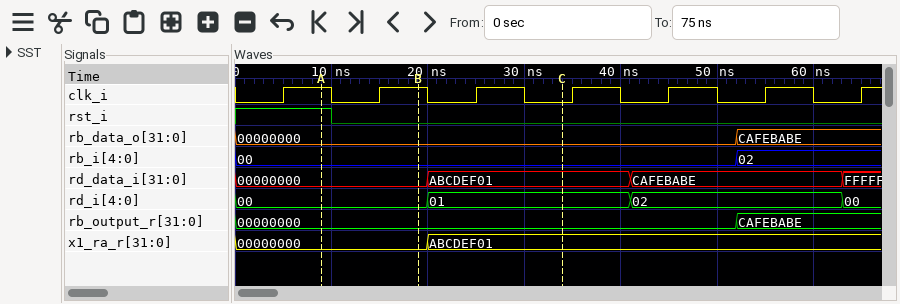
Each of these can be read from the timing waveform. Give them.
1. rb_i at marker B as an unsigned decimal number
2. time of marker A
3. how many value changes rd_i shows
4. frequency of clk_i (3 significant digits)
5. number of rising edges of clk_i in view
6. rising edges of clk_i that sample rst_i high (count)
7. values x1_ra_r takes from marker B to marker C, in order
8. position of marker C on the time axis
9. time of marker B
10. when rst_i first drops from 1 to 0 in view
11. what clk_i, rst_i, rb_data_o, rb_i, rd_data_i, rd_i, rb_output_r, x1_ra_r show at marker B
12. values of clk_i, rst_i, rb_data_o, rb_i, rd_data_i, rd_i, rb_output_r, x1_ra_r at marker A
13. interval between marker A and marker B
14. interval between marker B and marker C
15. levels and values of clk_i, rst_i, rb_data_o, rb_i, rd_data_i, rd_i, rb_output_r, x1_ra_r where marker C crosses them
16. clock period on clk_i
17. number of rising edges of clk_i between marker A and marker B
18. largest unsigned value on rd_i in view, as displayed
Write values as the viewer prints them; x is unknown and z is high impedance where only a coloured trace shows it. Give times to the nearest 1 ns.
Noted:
0
9 ns
3
100 MHz
7
1
00000000, ABCDEF01
34 ns
19 ns
10 ns
clk_i=1, rst_i=0, rb_data_o=00000000, rb_i=00, rd_data_i=00000000, rd_i=00, rb_output_r=00000000, x1_ra_r=00000000
clk_i=1, rst_i=1, rb_data_o=00000000, rb_i=00, rd_data_i=00000000, rd_i=00, rb_output_r=00000000, x1_ra_r=00000000
10 ns
15 ns
clk_i=0, rst_i=0, rb_data_o=00000000, rb_i=00, rd_data_i=ABCDEF01, rd_i=01, rb_output_r=00000000, x1_ra_r=ABCDEF01
10 ns
1
02
